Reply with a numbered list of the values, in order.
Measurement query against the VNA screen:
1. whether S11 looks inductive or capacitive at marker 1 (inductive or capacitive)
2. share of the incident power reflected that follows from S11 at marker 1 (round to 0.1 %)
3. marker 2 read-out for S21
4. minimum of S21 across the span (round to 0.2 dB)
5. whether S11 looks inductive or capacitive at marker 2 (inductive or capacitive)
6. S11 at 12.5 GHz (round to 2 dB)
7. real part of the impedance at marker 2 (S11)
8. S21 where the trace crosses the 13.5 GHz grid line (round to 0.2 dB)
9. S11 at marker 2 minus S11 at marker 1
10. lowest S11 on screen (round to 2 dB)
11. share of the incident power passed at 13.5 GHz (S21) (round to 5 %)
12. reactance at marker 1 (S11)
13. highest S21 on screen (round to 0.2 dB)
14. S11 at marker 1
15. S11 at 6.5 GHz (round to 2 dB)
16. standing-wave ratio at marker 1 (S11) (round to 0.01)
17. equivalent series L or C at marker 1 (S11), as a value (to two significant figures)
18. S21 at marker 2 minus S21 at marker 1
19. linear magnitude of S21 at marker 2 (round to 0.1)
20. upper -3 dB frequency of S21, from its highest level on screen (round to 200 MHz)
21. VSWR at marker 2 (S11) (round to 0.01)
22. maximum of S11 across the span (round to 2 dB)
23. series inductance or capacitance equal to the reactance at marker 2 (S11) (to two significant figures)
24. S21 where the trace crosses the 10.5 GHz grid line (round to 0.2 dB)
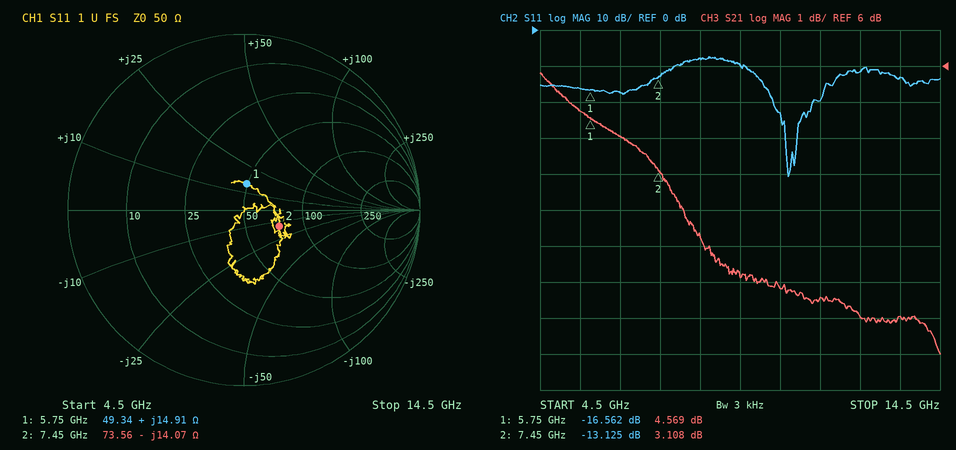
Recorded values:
1. inductive
2. 2.2 %
3. 3.108 dB
4. -2.0 dB
5. capacitive
6. -12 dB
7. 73.56 Ω
8. -1.0 dB
9. 3.437 dB
10. -40 dB
11. 80 %
12. +14.91 Ω
13. 5.8 dB
14. -16.562 dB
15. -18 dB
16. 1.35
17. 410 pH
18. -1.461 dB
19. 1.4
20. 7.6 GHz
21. 1.57
22. -8 dB
23. 1.5 pF
24. -0.2 dB
